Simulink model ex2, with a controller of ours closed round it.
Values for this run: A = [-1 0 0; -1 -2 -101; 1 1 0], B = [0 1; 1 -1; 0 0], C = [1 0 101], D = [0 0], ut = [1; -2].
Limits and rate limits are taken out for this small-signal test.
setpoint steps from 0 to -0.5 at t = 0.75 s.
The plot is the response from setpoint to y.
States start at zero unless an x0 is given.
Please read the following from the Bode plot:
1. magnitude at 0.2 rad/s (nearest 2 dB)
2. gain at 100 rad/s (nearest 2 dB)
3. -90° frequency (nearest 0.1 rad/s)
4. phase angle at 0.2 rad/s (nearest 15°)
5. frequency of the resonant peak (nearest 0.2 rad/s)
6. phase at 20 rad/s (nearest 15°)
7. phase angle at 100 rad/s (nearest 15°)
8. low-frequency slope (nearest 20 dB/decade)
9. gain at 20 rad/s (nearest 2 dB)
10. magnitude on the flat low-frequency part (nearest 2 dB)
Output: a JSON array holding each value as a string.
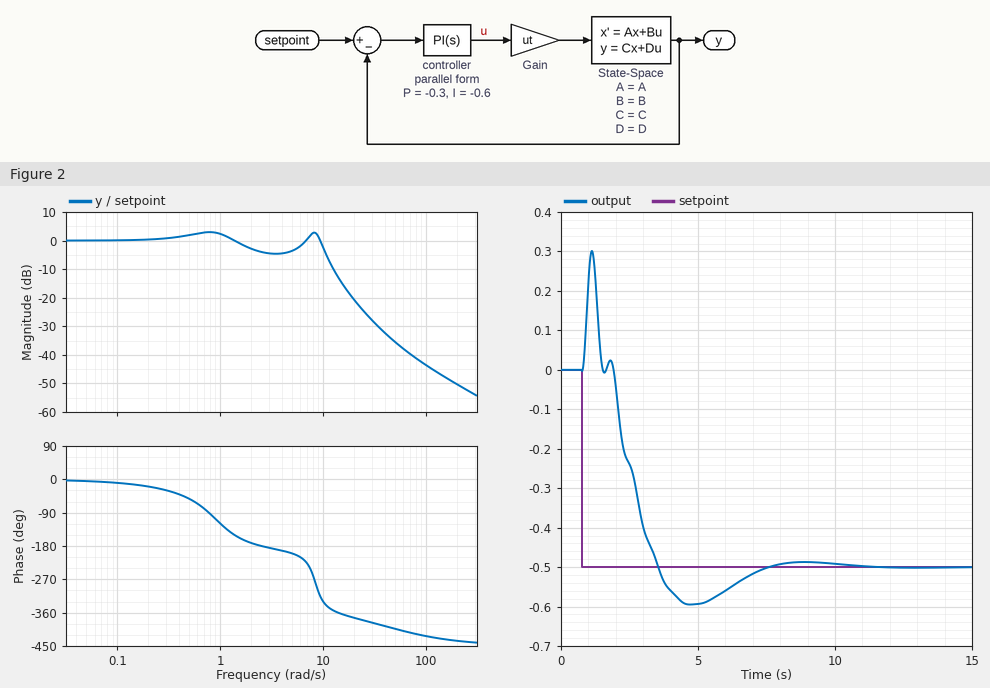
["0 dB", "-44 dB", "0.8 rad/s", "-15°", "0.8 rad/s", "-375°", "-420°", "0 dB/decade", "-20 dB", "0 dB"]
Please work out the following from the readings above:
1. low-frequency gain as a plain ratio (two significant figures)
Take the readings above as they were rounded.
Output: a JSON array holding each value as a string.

["1.0"]
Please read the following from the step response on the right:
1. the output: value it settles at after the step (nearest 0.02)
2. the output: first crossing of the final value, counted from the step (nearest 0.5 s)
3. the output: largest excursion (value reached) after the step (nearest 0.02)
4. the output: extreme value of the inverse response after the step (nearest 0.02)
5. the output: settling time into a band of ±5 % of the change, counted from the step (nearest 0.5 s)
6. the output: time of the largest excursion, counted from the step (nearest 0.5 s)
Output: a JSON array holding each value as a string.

["-0.50", "3.0 s", "-0.60", "0.30", "6.0 s", "4.0 s"]
